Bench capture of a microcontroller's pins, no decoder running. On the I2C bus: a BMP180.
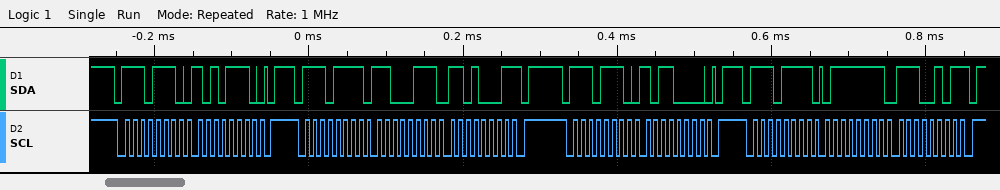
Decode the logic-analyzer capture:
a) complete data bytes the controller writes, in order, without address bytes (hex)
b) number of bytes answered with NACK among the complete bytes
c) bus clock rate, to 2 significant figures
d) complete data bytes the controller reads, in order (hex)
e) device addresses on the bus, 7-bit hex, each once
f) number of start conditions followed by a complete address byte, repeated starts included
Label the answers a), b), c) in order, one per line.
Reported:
a) AE B0
b) 2
c) 100 kHz
d) C7 D1 7F E5
e) 0x77
f) 4
